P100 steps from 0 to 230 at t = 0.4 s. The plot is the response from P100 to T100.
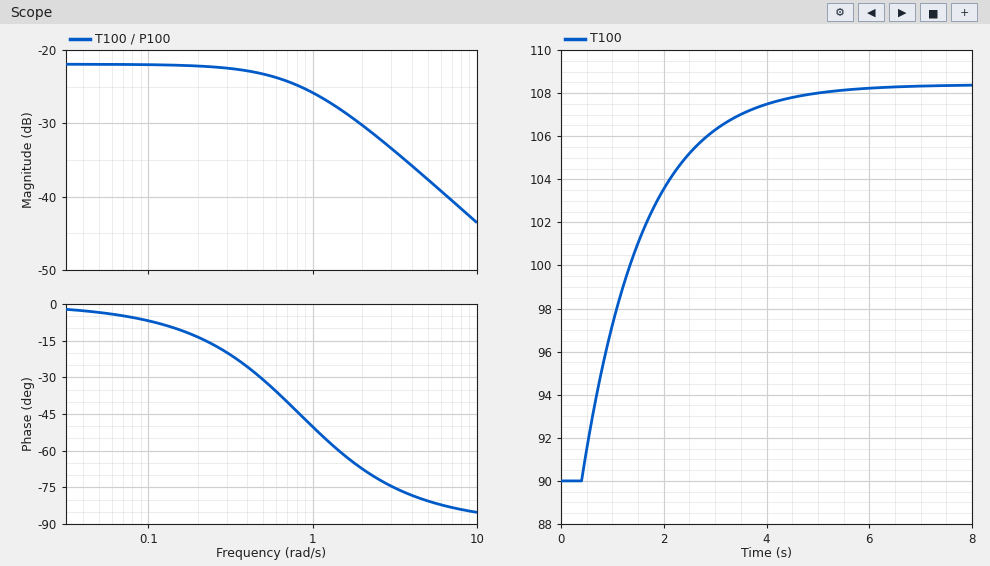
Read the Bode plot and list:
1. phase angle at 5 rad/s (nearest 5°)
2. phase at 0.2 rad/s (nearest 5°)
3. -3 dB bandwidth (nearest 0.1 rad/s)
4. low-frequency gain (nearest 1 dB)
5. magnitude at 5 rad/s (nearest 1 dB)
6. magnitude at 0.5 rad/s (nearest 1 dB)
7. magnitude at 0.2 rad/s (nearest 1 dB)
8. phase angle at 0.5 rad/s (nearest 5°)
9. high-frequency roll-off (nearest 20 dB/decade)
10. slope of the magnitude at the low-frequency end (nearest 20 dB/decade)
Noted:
-80°
-15°
0.8 rad/s
-22 dB
-38 dB
-23 dB
-22 dB
-30°
-20 dB/decade
0 dB/decade
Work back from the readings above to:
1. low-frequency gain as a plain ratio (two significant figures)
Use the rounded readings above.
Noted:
0.079
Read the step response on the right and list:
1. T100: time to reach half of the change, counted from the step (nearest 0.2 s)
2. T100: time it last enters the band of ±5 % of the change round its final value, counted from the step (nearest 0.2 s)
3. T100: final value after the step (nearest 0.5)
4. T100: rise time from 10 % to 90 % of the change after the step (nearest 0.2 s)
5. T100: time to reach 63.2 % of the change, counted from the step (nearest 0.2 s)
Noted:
0.8 s
3.6 s
108.5
2.6 s
1.2 s
